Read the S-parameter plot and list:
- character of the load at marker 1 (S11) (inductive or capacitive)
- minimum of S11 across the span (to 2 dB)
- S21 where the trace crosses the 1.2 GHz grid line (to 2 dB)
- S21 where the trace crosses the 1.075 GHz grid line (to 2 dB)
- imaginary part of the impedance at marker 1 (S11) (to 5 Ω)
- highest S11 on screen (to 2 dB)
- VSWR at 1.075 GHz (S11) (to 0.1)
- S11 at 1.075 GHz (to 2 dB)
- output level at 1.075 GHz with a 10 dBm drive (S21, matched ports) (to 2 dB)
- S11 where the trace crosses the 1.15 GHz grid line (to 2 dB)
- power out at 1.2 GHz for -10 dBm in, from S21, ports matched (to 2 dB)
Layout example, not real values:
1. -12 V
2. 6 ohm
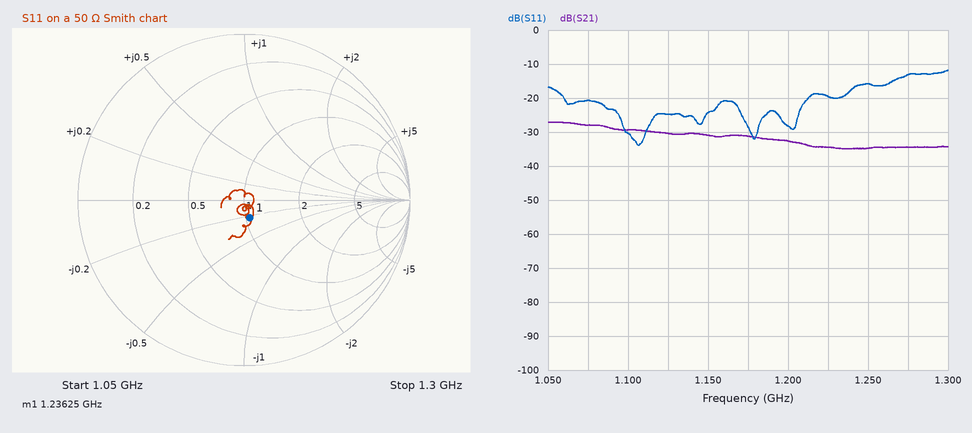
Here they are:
1. capacitive
2. -34 dB
3. -32 dB
4. -28 dB
5. -10 Ω
6. -12 dB
7. 1.2
8. -20 dB
9. -18 dBm
10. -24 dB
11. -42 dBm
